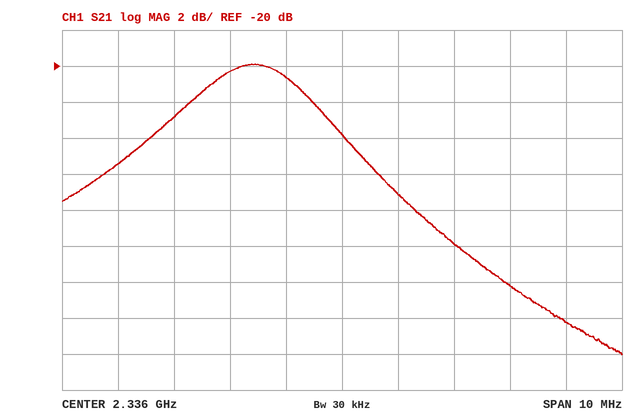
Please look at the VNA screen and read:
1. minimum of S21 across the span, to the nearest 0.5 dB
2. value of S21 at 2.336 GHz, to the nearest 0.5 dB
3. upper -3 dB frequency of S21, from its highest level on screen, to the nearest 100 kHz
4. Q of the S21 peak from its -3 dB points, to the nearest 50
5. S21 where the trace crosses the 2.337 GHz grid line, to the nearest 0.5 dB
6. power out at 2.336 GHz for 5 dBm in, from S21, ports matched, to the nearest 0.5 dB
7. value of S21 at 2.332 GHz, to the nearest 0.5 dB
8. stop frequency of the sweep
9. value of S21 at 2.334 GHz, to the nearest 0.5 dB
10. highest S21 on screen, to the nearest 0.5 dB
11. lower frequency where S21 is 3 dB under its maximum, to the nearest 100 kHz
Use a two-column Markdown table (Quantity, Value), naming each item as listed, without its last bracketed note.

| Quantity | Value |
|---|---|
| minimum of S21 across the span, to the nearest 0.5 dB | -36.0 dB |
| value of S21 at 2.336 GHz, to the nearest 0.5 dB | -24.0 dB |
| upper -3 dB frequency of S21, from its highest level on screen, to the nearest 100 kHz | 2.3357 GHz |
| Q of the S21 peak from its -3 dB points, to the nearest 50 | 850 |
| S21 where the trace crosses the 2.337 GHz grid line, to the nearest 0.5 dB | -27.0 dB |
| power out at 2.336 GHz for 5 dBm in, from S21, ports matched, to the nearest 0.5 dB | -19.0 dBm |
| value of S21 at 2.332 GHz, to the nearest 0.5 dB | -25.5 dB |
| stop frequency of the sweep | 2.341 GHz |
| value of S21 at 2.334 GHz, to the nearest 0.5 dB | -20.5 dB |
| highest S21 on screen, to the nearest 0.5 dB | -20.0 dB |
| lower frequency where S21 is 3 dB under its maximum, to the nearest 100 kHz | 2.3330 GHz |
